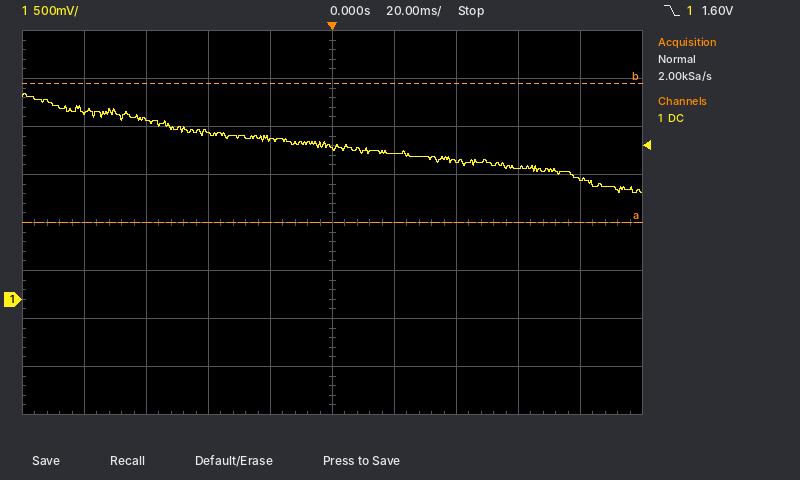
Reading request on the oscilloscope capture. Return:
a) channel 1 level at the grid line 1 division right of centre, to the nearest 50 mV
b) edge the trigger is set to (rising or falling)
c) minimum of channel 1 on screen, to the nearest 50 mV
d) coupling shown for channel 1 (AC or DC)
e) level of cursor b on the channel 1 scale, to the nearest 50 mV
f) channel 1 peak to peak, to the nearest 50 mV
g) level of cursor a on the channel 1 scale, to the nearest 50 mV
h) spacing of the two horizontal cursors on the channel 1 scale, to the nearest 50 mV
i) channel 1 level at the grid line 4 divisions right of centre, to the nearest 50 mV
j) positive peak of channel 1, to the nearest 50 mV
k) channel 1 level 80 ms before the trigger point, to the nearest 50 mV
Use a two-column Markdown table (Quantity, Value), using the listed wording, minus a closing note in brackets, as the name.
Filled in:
| Quantity | Value |
|---|---|
| channel 1 level at the grid line 1 division right of centre, to the nearest 50 mV | 1.50 V |
| edge the trigger is set to | falling |
| minimum of channel 1 on screen, to the nearest 50 mV | 1.10 V |
| coupling shown for channel 1 | DC |
| level of cursor b on the channel 1 scale, to the nearest 50 mV | 2.25 V |
| channel 1 peak to peak, to the nearest 50 mV | 1.05 V |
| level of cursor a on the channel 1 scale, to the nearest 50 mV | 800 mV |
| spacing of the two horizontal cursors on the channel 1 scale, to the nearest 50 mV | 1.45 V |
| channel 1 level at the grid line 4 divisions right of centre, to the nearest 50 mV | 1.25 V |
| positive peak of channel 1, to the nearest 50 mV | 2.15 V |
| channel 1 level 80 ms before the trigger point, to the nearest 50 mV | 1.95 V |
